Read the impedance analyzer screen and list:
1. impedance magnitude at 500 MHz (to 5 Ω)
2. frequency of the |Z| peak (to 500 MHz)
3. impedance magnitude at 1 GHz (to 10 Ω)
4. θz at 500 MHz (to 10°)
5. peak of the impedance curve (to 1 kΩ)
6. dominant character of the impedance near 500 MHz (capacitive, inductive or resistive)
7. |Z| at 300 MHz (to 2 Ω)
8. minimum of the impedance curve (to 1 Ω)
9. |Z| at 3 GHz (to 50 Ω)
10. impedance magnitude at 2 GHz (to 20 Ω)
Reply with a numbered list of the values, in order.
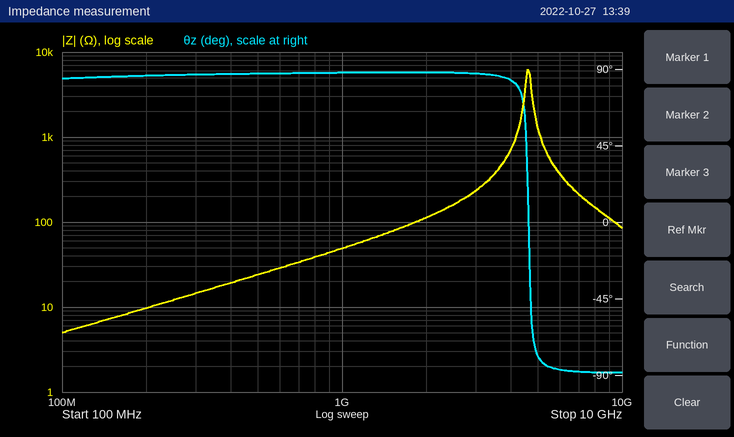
1. 25 Ω
2. 4.5 GHz
3. 50 Ω
4. 90°
5. 6 kΩ
6. inductive
7. 14 Ω
8. 5 Ω
9. 250 Ω
10. 120 Ω
